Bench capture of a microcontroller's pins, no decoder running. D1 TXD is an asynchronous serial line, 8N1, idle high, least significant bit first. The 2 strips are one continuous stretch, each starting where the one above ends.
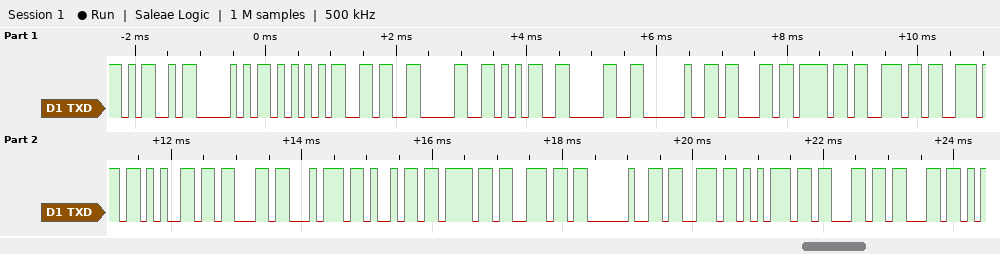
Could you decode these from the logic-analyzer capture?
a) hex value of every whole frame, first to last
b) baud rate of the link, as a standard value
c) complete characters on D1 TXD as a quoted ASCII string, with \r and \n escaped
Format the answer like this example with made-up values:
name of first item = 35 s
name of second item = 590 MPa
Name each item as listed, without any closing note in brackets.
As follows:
hex value of every whole frame, first to last = 4D 50 55 36 30 35 30 20 63 6F 6E 6E 65 63 74 69 6F 6E 20 73 75 63 63
baud rate of the link, as a standard value = 9600 baud
complete characters on D1 TXD as a quoted ASCII string, with \r and \n escaped = "MPU6050 connection succ"
